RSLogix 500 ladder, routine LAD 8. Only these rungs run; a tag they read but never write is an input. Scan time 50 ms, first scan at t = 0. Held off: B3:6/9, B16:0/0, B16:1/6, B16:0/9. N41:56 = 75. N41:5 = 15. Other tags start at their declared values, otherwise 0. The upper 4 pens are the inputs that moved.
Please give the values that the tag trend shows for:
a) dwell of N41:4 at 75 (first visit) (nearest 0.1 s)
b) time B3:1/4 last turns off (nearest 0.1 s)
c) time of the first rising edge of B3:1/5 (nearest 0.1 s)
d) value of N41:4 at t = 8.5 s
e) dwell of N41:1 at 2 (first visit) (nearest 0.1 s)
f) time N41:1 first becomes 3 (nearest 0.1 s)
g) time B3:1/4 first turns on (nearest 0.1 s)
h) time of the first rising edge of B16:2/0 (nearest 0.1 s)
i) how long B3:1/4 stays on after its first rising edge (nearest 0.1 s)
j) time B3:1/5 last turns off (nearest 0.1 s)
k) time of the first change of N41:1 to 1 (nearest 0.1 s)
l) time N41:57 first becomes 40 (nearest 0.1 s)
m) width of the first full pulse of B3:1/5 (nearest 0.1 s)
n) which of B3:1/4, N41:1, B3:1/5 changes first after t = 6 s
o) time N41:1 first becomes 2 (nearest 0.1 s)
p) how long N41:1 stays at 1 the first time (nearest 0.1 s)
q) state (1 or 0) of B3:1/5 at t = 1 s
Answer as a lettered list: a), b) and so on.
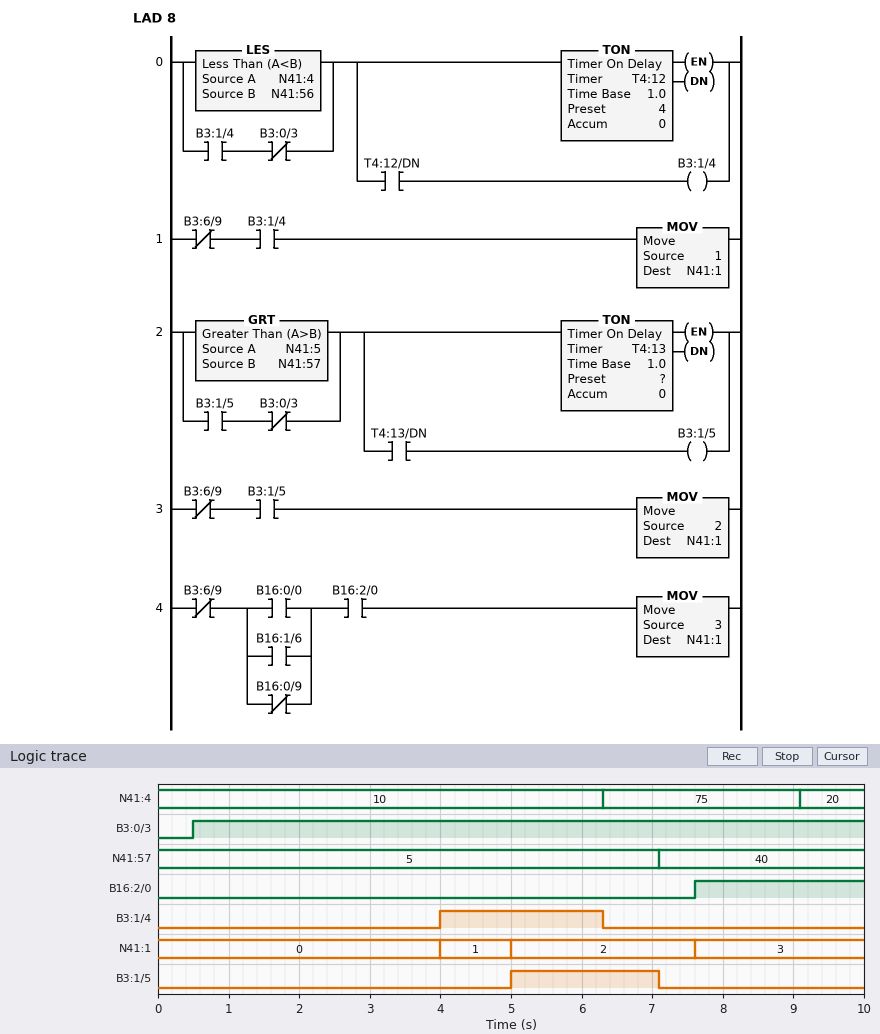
a) 2.8 s
b) 6.3 s
c) 5.0 s
d) 75
e) 2.6 s
f) 7.6 s
g) 4.0 s
h) 7.6 s
i) 2.3 s
j) 7.1 s
k) 4.0 s
l) 7.1 s
m) 2.1 s
n) B3:1/4
o) 5.0 s
p) 1.0 s
q) 0
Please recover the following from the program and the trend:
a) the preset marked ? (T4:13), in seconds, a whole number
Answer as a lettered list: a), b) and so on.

a) 5 s
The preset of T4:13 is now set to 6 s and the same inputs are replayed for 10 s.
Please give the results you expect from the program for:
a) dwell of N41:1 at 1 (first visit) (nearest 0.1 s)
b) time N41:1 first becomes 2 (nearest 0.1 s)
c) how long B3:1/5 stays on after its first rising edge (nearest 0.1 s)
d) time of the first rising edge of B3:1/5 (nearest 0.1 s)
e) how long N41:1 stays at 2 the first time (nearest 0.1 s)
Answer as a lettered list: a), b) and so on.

a) 2.0 s
b) 6.0 s
c) 1.1 s
d) 6.0 s
e) 1.6 s
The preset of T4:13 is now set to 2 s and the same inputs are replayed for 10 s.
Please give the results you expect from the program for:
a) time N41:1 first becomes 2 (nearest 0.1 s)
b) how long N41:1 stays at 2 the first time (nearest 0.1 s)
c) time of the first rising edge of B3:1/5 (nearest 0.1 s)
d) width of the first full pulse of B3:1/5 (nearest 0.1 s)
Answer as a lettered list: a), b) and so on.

a) 2.0 s
b) 5.6 s
c) 2.0 s
d) 5.1 s
